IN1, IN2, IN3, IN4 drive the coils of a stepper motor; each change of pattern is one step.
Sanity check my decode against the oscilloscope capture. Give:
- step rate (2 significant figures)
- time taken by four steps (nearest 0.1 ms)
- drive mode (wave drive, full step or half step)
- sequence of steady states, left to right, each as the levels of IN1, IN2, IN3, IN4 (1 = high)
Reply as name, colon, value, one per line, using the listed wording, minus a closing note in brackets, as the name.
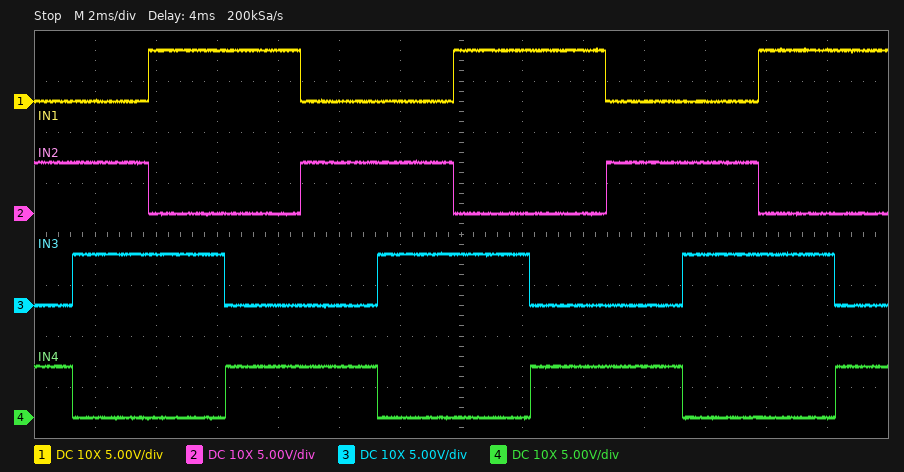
step rate: 400 steps/s
time taken by four steps: 10.0 ms
drive mode: full step
sequence of steady states, left to right, each as the levels of IN1, IN2, IN3, IN4: 0101 0110 1010 1001 0101 0110 1010 1001 0101 0110 1010 1001
